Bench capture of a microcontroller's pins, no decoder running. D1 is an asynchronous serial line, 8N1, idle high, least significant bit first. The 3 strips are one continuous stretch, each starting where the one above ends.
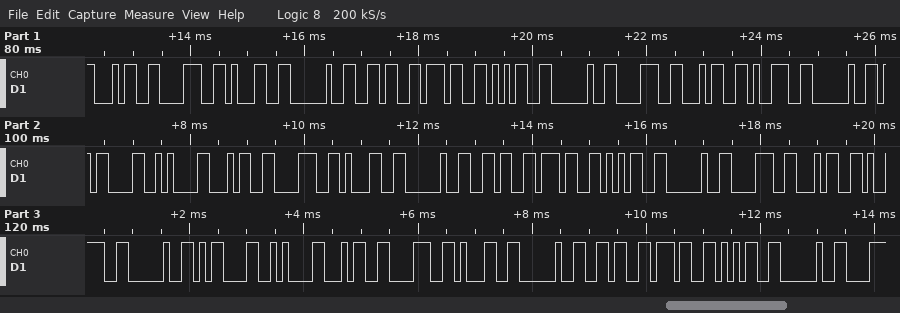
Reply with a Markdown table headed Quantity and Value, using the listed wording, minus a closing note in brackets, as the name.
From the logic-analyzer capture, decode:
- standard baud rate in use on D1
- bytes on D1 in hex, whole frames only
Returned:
| Quantity | Value |
|---|---|
| standard baud rate in use on D1 | 9600 baud |
| bytes on D1 in hex, whole frames only | 34 38 31 20 36 37 35 20 38 34 39 20 0D 0A 34 38 31 20 36 37 35 20 38 34 39 20 0D 0A 34 38 31 20 36 37 35 20 |
